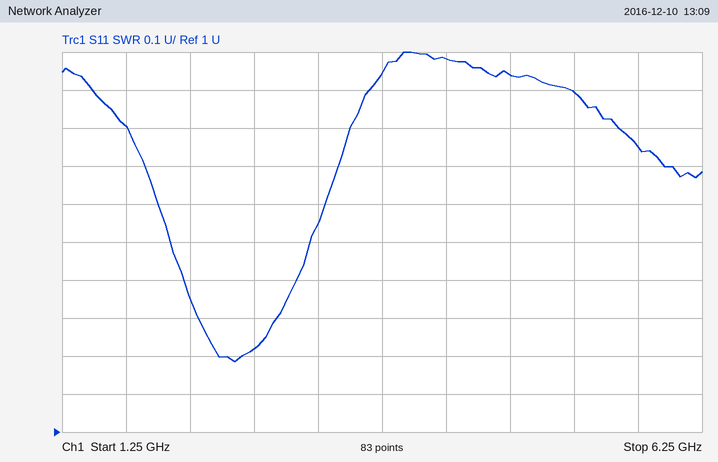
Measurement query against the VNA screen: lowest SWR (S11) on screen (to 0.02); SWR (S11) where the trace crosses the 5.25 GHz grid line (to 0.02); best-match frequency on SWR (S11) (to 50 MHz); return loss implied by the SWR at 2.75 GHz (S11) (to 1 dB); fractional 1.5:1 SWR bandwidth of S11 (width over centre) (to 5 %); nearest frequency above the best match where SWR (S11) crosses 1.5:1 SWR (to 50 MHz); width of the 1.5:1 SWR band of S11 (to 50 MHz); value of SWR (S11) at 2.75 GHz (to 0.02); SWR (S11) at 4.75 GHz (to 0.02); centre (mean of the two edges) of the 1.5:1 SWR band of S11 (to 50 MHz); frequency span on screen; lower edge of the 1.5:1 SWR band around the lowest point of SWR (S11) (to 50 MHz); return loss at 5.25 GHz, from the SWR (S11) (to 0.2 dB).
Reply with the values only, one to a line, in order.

1.18
1.90
2.60 GHz
20 dB
40 %
3.20 GHz
1.10 GHz
1.22
1.94
2.65 GHz
5 GHz
2.10 GHz
10.2 dB
